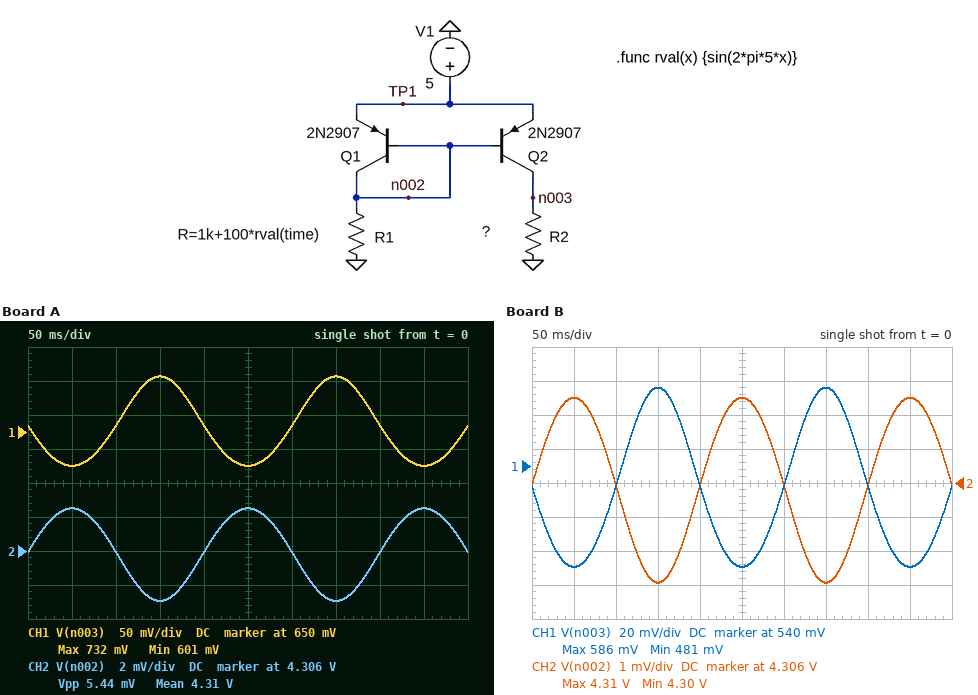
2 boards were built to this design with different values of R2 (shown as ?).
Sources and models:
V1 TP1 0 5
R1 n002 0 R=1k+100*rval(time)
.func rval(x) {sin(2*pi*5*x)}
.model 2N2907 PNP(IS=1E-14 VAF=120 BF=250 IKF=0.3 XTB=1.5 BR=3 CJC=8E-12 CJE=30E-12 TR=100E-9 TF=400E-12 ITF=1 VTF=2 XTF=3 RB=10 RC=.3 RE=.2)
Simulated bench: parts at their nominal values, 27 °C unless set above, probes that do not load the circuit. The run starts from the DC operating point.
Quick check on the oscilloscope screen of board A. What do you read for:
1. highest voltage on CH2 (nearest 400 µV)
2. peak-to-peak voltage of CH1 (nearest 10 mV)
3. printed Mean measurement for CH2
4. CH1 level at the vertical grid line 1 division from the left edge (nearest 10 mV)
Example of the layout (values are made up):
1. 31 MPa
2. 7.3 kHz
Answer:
1. 4.3084 V
2. 130 mV
3. 4.31 V
4. 600 mV
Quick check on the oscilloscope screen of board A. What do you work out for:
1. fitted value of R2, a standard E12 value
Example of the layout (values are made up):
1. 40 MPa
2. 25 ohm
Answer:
1. 150 Ω
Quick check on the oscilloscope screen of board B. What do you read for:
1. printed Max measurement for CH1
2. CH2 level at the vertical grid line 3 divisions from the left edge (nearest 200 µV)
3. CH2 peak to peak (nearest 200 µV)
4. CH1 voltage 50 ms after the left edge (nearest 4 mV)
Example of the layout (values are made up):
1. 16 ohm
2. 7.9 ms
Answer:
1. 586 mV
2. 4.3030 V
3. 5.4 mV
4. 480 mV
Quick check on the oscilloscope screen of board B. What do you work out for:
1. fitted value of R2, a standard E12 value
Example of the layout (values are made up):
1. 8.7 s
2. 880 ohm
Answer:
1. 120 Ω
